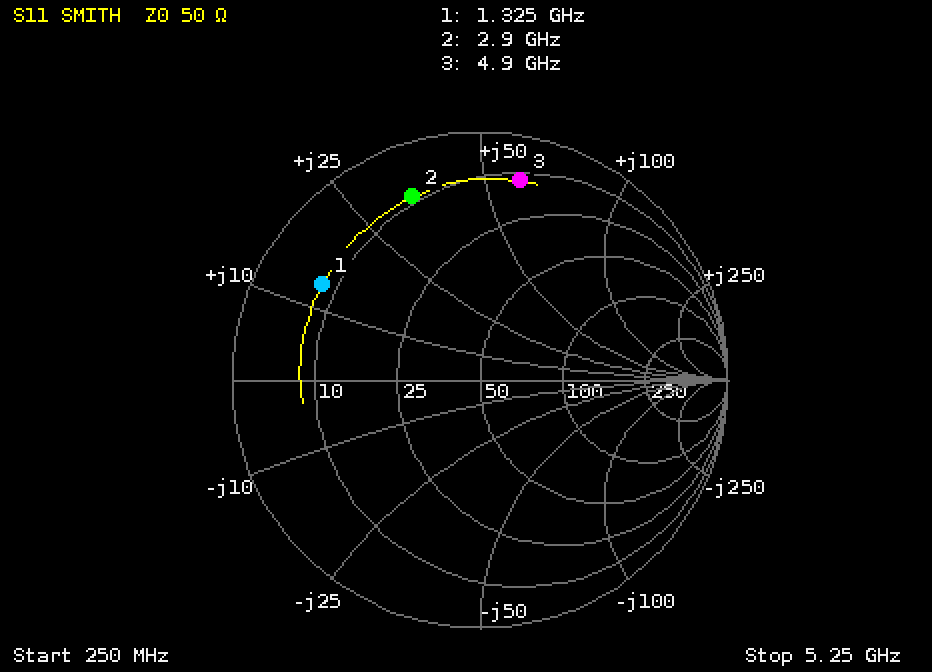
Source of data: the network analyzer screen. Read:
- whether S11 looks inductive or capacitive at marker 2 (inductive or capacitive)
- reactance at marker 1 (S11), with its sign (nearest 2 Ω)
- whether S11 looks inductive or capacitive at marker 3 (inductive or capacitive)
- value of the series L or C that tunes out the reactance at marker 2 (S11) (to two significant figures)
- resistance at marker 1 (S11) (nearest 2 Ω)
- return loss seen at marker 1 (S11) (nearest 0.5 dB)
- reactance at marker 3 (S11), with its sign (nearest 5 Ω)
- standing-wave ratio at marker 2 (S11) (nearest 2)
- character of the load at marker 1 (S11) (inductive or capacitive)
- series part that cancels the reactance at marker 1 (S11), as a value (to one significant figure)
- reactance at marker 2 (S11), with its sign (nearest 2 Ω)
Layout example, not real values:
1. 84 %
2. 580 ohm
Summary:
1. inductive
2. +14 Ω
3. inductive
4. 1.6 pF
5. 8 Ω
6. 2.5 dB
7. +60 Ω
8. 8
9. inductive
10. 9 pF
11. +34 Ω
